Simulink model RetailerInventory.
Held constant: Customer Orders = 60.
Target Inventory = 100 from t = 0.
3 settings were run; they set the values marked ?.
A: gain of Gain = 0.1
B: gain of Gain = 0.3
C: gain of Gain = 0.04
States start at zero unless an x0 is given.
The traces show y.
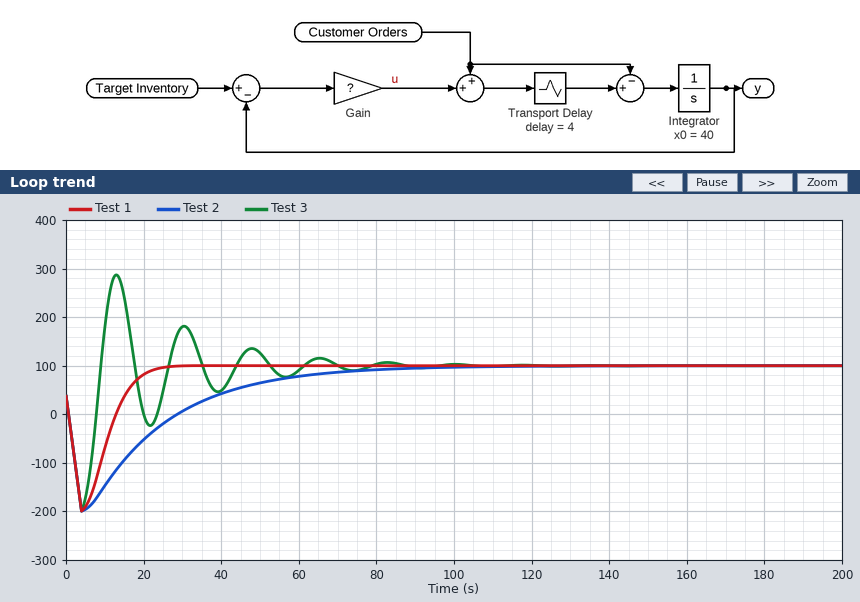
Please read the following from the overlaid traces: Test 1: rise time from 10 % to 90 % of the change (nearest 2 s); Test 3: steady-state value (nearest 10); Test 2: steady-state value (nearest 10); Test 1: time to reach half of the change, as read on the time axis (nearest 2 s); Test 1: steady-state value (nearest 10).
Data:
8 s
100
100
18 s
100
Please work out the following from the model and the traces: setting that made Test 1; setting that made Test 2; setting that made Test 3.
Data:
A
C
B
